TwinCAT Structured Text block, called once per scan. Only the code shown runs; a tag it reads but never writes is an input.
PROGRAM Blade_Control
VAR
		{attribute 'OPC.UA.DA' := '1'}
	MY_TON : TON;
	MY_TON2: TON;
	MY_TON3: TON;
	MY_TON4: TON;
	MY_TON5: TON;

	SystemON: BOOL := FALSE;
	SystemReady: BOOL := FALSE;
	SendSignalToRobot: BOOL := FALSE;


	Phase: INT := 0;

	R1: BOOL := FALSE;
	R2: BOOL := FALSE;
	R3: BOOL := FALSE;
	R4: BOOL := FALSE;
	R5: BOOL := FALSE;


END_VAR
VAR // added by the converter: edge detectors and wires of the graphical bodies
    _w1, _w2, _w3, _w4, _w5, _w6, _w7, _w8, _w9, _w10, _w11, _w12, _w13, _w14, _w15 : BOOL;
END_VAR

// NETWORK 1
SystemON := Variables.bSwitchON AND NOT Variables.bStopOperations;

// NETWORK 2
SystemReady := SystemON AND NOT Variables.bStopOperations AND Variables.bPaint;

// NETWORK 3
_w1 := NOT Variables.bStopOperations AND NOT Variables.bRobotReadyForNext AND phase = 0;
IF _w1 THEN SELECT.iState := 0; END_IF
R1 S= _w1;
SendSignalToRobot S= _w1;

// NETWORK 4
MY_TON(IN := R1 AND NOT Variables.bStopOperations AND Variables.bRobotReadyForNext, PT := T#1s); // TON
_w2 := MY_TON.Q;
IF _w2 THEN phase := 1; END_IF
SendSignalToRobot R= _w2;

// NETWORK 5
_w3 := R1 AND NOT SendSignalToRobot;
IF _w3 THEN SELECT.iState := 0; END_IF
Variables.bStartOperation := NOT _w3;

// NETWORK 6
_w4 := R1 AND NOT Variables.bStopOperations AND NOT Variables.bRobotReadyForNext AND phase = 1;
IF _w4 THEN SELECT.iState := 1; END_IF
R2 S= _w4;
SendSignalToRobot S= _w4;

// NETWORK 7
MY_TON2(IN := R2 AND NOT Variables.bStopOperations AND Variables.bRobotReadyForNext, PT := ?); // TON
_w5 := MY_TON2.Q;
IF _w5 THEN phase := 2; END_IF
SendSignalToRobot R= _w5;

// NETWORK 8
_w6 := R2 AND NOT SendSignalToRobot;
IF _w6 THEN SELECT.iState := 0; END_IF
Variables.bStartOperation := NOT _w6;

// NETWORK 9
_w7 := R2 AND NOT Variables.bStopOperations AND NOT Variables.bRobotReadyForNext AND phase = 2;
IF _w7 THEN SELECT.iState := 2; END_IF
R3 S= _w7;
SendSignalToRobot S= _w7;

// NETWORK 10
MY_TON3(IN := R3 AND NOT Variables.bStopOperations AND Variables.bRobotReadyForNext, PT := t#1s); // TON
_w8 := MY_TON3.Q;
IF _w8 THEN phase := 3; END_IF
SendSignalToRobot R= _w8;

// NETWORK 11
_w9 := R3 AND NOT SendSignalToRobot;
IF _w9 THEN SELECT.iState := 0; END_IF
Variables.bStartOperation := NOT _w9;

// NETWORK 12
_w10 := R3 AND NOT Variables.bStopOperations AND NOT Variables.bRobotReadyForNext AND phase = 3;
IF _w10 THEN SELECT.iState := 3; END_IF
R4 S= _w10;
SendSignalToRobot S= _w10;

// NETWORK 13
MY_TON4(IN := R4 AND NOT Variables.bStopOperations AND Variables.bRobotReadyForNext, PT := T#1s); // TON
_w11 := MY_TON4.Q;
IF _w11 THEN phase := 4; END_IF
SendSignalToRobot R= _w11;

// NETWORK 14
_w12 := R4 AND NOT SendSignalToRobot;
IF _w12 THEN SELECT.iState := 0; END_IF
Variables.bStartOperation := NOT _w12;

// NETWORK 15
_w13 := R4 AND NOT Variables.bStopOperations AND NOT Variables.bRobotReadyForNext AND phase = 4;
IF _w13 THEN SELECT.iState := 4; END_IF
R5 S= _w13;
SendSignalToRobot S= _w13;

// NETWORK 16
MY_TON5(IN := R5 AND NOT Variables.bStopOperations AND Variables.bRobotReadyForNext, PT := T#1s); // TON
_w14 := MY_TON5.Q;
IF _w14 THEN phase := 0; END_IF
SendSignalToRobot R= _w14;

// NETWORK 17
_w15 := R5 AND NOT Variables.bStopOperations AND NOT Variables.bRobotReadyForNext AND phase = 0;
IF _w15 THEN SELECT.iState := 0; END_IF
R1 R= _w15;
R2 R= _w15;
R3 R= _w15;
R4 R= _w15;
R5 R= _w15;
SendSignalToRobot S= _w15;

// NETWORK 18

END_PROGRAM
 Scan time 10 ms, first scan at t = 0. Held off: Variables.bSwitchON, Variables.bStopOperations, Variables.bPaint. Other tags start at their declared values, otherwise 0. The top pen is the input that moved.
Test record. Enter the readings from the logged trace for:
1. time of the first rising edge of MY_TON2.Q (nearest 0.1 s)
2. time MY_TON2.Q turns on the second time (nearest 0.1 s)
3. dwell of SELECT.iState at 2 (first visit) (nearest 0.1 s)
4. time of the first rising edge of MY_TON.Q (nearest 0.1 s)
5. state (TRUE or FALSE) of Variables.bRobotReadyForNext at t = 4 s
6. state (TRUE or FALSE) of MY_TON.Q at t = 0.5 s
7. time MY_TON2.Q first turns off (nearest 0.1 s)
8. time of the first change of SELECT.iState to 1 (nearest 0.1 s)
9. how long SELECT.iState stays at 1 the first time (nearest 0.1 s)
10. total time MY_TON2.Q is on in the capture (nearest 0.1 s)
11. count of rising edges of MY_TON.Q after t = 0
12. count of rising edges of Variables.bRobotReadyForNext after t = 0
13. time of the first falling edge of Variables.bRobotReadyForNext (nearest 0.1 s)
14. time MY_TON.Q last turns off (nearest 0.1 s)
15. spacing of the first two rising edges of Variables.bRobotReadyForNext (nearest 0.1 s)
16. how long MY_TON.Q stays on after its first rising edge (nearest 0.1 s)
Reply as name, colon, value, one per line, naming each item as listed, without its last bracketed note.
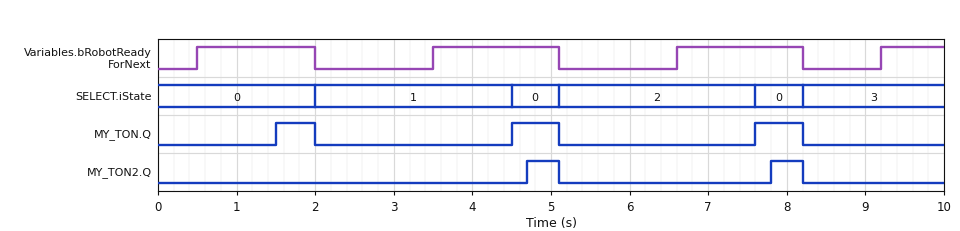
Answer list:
time of the first rising edge of MY_TON2.Q: 4.7 s
time MY_TON2.Q turns on the second time: 7.8 s
dwell of SELECT.iState at 2 (first visit): 2.5 s
time of the first rising edge of MY_TON.Q: 1.5 s
state (TRUE or FALSE) of Variables.bRobotReadyForNext at t = 4 s: TRUE
state (TRUE or FALSE) of MY_TON.Q at t = 0.5 s: FALSE
time MY_TON2.Q first turns off: 5.1 s
time of the first change of SELECT.iState to 1: 2.0 s
how long SELECT.iState stays at 1 the first time: 2.5 s
total time MY_TON2.Q is on in the capture: 0.8 s
count of rising edges of MY_TON.Q after t = 0: 3
count of rising edges of Variables.bRobotReadyForNext after t = 0: 4
time of the first falling edge of Variables.bRobotReadyForNext: 2.0 s
time MY_TON.Q last turns off: 8.2 s
spacing of the first two rising edges of Variables.bRobotReadyForNext: 3.0 s
how long MY_TON.Q stays on after its first rising edge: 0.5 s
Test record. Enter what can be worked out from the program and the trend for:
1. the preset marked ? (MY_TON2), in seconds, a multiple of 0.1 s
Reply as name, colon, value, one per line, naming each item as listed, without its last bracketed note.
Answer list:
the preset marked ? (MY_TON2), in seconds, a multiple of 0.1 s: 1.2 s
